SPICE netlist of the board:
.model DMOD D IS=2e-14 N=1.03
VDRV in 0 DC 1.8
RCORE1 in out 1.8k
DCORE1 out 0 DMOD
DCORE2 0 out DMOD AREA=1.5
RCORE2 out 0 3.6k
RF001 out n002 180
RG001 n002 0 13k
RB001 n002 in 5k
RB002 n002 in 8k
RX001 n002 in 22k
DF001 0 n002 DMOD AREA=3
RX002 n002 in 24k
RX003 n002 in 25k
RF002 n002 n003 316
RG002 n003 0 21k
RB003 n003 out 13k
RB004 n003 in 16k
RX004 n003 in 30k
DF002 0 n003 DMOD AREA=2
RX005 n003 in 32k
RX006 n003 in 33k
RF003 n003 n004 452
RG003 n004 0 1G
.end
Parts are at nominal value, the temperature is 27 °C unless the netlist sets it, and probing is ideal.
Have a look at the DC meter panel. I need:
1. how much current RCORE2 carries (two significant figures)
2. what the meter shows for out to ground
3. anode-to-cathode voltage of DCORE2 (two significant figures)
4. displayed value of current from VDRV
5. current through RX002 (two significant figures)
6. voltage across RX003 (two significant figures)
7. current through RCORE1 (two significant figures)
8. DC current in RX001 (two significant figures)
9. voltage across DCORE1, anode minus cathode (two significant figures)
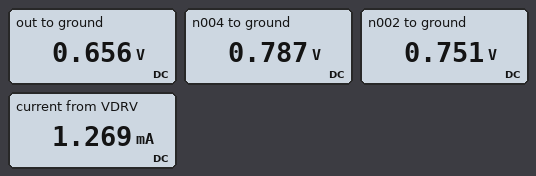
180 µA
0.656 V
-660 mV
1.269 mA
44 µA
1.0 V
640 µA
48 µA
660 mV
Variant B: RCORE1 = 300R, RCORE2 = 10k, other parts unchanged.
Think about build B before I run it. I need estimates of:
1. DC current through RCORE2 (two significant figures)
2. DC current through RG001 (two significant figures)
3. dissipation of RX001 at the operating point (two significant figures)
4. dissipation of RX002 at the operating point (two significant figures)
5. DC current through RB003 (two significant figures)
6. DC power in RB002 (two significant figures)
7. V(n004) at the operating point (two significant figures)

69 µA
60 µA
47 µW
43 µW
9.6 µA
130 µW
820 mV
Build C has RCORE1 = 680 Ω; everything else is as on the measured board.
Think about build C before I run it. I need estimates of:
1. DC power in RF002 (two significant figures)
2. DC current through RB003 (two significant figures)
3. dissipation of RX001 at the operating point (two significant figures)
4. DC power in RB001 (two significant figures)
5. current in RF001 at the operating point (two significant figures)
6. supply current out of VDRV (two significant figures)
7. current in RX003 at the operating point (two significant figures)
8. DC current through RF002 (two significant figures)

3.8 µW
9.8 µA
48 µW
210 µW
520 µA
2.3 mA
41 µA
110 µA
